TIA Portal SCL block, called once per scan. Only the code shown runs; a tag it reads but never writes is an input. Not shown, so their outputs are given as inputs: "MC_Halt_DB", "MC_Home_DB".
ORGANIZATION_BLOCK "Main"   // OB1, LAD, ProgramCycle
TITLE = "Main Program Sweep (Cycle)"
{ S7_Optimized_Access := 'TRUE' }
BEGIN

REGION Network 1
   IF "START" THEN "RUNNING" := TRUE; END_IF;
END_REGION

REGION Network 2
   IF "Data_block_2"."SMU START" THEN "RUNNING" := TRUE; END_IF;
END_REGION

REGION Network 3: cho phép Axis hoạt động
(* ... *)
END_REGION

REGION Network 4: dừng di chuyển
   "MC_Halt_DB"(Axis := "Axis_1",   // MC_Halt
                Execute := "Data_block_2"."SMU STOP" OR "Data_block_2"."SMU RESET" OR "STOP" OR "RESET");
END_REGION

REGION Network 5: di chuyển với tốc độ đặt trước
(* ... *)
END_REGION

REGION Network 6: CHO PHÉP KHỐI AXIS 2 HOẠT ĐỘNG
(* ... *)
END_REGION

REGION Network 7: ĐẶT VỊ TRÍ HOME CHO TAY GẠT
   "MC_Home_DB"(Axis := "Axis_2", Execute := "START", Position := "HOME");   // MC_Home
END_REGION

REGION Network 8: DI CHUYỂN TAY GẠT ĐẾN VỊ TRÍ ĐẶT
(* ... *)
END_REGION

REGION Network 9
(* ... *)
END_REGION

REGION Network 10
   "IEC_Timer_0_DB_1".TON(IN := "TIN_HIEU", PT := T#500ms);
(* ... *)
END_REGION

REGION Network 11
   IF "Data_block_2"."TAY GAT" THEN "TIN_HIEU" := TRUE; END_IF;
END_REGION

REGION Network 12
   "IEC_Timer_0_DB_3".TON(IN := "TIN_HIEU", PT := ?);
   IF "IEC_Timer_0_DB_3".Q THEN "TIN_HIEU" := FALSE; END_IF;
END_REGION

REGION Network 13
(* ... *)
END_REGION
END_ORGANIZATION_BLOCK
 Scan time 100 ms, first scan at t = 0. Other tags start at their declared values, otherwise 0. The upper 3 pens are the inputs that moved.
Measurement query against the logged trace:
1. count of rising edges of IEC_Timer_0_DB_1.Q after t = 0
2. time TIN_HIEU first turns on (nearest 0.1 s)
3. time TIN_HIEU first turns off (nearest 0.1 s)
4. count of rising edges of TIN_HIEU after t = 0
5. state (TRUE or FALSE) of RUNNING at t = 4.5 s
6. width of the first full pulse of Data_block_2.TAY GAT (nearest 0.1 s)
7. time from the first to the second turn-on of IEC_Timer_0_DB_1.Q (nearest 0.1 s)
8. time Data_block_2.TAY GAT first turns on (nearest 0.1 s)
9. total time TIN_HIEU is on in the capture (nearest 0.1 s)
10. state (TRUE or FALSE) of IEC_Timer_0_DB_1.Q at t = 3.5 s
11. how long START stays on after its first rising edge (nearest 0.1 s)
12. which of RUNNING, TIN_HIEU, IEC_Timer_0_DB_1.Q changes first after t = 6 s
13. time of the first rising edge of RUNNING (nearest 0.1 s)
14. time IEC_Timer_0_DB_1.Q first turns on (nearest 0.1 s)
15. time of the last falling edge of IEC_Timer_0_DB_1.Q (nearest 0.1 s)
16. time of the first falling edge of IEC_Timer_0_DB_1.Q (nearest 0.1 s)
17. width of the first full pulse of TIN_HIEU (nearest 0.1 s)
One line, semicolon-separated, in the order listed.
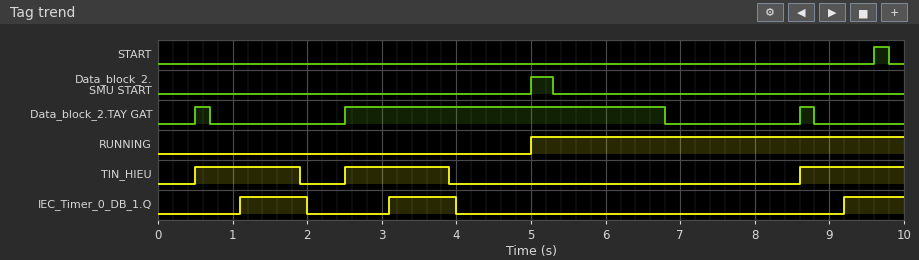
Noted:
3; 0.5 s; 1.9 s; 3; FALSE; 0.2 s; 2.0 s; 0.5 s; 4.2 s; TRUE; 0.2 s; TIN_HIEU; 5.0 s; 1.1 s; 4.0 s; 2.0 s; 1.4 s
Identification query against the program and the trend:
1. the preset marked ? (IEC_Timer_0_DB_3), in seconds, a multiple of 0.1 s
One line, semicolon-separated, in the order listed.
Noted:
1.4 s
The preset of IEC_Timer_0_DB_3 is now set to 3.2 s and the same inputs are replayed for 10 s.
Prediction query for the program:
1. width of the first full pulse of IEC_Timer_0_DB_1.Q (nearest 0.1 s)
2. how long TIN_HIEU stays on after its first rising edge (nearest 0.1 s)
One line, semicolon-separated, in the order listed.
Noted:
2.7 s; 3.2 s
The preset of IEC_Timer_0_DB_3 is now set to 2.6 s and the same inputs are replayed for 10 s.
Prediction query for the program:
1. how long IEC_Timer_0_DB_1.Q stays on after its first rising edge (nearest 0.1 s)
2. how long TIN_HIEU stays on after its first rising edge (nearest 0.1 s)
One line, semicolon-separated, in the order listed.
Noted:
2.1 s; 2.6 s
